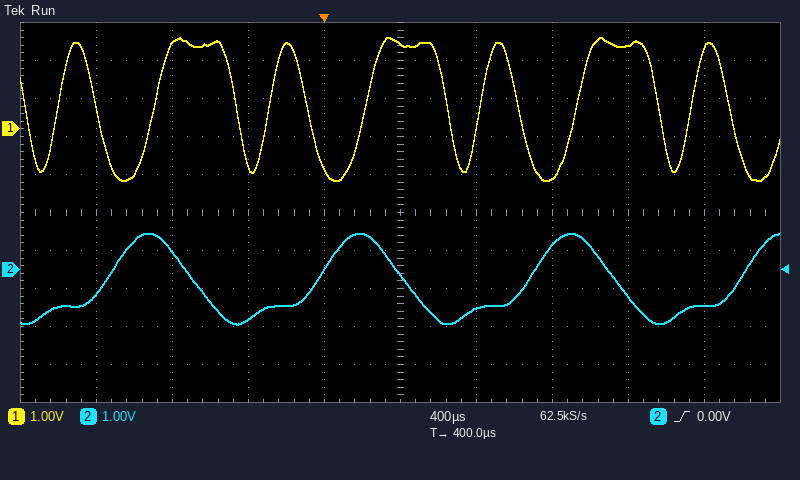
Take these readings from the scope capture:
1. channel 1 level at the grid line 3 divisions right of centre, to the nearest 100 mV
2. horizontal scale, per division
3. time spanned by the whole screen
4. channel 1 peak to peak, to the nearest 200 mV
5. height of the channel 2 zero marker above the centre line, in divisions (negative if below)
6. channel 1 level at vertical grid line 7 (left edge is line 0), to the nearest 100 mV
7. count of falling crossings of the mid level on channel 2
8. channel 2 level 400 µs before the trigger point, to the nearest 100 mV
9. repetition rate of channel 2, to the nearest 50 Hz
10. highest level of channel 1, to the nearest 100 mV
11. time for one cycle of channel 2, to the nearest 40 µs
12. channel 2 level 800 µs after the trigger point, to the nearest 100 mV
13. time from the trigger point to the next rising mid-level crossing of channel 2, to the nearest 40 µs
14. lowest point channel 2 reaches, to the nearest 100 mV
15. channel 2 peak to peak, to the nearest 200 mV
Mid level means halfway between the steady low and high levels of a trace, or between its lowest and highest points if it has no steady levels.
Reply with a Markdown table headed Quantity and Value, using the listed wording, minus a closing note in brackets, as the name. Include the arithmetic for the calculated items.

| Quantity | Value |
|---|---|
| channel 1 level at the grid line 3 divisions right of centre, to the nearest 100 mV | 2.2 V |
| horizontal scale, per division | 400 µs |
| time spanned by the whole screen | 4 ms |
| channel 1 peak to peak, to the nearest 200 mV | 3.8 V |
| height of the channel 2 zero marker above the centre line, in divisions | -1.5 div |
| channel 1 level at vertical grid line 7 (left edge is line 0), to the nearest 100 mV | -1.3 V |
| count of falling crossings of the mid level on channel 2 | 3 |
| channel 2 level 400 µs before the trigger point, to the nearest 100 mV | -1.3 V |
| repetition rate of channel 2, to the nearest 50 Hz | 1 / 1.12 ms ≈ 893 Hz, so 900 Hz to the nearest 50 Hz |
| highest level of channel 1, to the nearest 100 mV | 2.4 V |
| time for one cycle of channel 2, to the nearest 40 µs | 1.12 ms |
| channel 2 level 800 µs after the trigger point, to the nearest 100 mV | -1.0 V |
| time from the trigger point to the next rising mid-level crossing of channel 2, to the nearest 40 µs | 1.08 ms |
| lowest point channel 2 reaches, to the nearest 100 mV | -1.4 V |
| channel 2 peak to peak, to the nearest 200 mV | 2.4 V |
